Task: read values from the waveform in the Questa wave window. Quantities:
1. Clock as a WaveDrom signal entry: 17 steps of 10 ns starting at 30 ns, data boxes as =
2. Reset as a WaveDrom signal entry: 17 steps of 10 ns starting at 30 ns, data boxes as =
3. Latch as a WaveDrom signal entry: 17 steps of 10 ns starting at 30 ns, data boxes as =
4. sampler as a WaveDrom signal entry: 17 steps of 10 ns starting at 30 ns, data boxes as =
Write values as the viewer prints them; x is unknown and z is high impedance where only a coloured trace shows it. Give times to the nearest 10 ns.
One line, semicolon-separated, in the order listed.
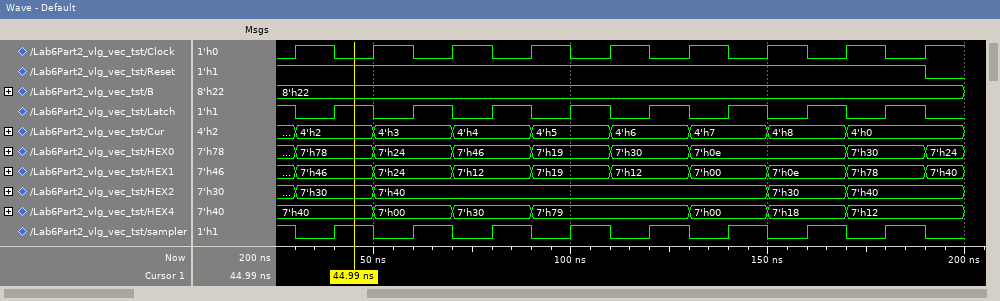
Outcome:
{name: 'Clock', wave: '10101010101010101'}; {name: 'Reset', wave: '1...............0'}; {name: 'Latch', wave: '01010101010101010'}; {name: 'sampler', wave: '01010101010101010'}
